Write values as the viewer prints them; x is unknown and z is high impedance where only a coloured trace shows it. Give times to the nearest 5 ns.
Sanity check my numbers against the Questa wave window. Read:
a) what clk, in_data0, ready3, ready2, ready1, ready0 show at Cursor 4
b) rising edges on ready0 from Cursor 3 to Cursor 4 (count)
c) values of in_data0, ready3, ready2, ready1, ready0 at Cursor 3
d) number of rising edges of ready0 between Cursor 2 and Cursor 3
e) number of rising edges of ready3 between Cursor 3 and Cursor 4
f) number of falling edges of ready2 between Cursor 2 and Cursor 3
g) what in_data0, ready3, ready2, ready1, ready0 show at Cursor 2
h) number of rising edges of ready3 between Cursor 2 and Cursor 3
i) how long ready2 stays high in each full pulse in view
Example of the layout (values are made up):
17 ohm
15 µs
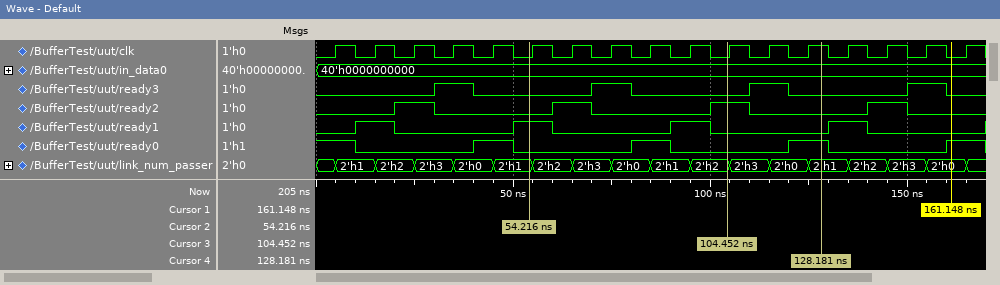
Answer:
clk=1, in_data0=40'h0000000000, ready3=0, ready2=0, ready1=0, ready0=1
1
in_data0=40'h0000000000, ready3=0, ready2=1, ready1=0, ready0=0
1
1
1
in_data0=40'h0000000000, ready3=0, ready2=0, ready1=1, ready0=0
1
10 ns, 10 ns, 10 ns, 10 ns
